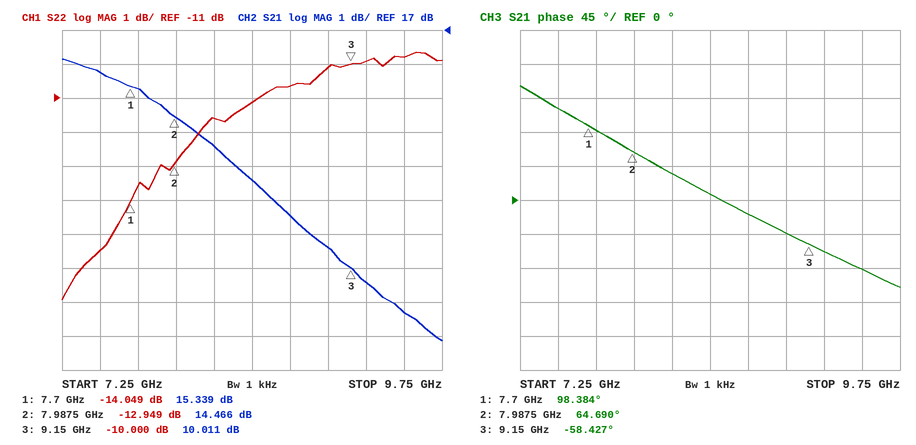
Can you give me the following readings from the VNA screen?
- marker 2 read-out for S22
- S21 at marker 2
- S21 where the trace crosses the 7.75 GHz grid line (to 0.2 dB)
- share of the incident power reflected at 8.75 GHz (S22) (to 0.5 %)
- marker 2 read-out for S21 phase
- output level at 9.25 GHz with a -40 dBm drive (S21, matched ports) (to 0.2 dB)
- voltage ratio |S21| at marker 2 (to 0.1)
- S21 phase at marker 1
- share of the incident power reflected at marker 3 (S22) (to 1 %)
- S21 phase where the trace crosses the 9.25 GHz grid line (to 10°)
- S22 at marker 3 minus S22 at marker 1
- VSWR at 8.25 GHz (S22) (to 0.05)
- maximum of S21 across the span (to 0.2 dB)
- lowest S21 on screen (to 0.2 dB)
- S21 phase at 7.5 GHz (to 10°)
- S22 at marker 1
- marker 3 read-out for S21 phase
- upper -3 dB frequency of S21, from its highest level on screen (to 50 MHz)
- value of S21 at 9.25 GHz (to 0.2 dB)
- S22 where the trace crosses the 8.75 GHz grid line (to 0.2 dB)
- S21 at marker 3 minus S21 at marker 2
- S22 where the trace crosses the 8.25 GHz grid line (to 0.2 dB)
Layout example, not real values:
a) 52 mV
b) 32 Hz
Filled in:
a) -12.949 dB
b) 14.466 dB
c) 15.2 dB
d) 8.5 %
e) 64.690°
f) -30.4 dBm
g) 5.3
h) 98.384°
i) 10 %
j) -70°
k) 4.049 dB
l) 1.70
m) 16.2 dB
n) 7.8 dB
o) 120°
p) -14.049 dB
q) -58.427°
r) 8.35 GHz
s) 9.6 dB
t) -10.6 dB
u) -4.455 dB
v) -11.6 dB
